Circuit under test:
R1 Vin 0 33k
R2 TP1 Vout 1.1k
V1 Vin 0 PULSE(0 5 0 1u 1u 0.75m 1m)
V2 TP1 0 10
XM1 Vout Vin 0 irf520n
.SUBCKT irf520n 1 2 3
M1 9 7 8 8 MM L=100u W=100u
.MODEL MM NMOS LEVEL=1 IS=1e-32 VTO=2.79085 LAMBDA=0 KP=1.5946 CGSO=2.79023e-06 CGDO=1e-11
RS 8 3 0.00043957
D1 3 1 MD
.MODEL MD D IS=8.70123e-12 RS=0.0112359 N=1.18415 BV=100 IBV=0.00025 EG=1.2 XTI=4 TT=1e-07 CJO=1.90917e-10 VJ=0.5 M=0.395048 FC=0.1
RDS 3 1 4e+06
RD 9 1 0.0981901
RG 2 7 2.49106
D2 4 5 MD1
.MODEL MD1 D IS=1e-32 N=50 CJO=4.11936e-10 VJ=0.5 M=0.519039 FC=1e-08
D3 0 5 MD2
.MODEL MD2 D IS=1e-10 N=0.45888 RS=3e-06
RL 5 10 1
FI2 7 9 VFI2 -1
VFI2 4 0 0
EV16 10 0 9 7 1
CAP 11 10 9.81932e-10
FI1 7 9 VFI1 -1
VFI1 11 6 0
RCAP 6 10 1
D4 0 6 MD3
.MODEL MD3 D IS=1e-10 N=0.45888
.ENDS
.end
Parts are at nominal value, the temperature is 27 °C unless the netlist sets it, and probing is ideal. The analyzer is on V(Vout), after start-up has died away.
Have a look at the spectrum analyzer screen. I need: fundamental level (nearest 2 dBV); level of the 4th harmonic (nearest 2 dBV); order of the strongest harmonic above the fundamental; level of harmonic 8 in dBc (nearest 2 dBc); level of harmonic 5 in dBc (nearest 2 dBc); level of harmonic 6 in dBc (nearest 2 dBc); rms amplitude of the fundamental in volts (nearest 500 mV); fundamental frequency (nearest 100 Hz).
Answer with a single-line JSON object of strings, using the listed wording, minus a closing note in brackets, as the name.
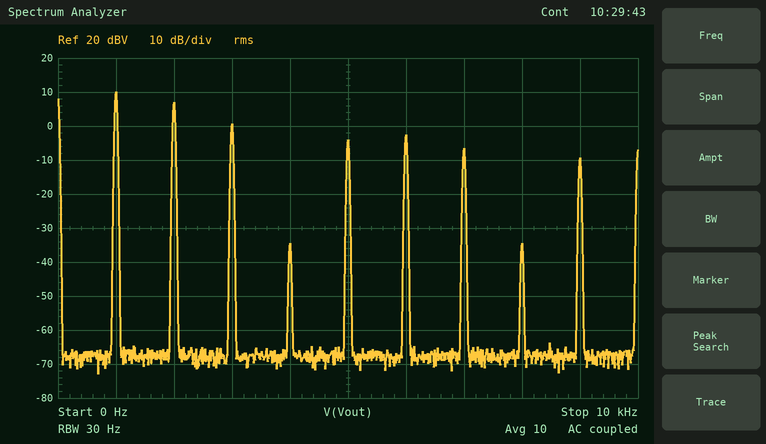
{"fundamental level": "10 dBV", "level of the 4th harmonic": "-34 dBV", "order of the strongest harmonic above the fundamental": "2", "level of harmonic 8 in dBc": "-44 dBc", "level of harmonic 5 in dBc": "-14 dBc", "level of harmonic 6 in dBc": "-12 dBc", "rms amplitude of the fundamental in volts": "3.0 V", "fundamental frequency": "1.0 kHz"}
